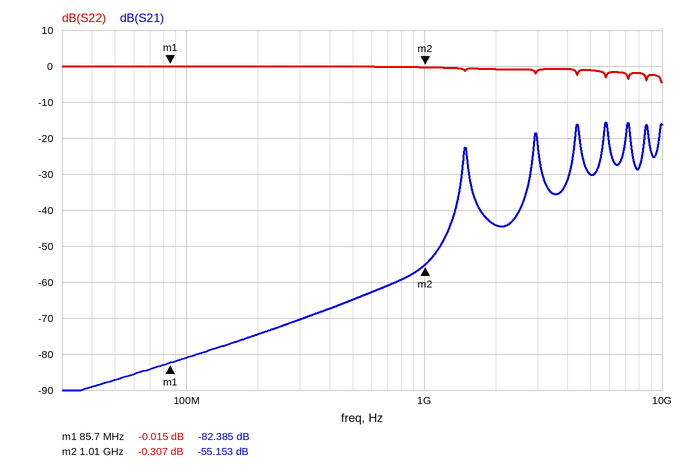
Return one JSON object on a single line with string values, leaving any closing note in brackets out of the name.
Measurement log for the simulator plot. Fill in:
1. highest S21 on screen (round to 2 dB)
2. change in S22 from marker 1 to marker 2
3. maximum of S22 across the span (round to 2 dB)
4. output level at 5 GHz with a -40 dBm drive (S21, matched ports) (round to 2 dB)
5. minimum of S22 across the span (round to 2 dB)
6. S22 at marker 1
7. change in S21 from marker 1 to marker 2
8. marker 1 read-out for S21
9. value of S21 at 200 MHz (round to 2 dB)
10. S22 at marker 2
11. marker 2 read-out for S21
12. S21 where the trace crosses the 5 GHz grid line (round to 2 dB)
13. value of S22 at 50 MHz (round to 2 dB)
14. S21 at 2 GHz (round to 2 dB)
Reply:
{"highest S21 on screen": "-16 dB", "change in S22 from marker 1 to marker 2": "-0.292 dB", "maximum of S22 across the span": "0 dB", "output level at 5 GHz with a -40 dBm drive (S21, matched ports)": "-70 dBm", "minimum of S22 across the span": "-4 dB", "S22 at marker 1": "-0.015 dB", "change in S21 from marker 1 to marker 2": "27.232 dB", "marker 1 read-out for S21": "-82.385 dB", "value of S21 at 200 MHz": "-74 dB", "S22 at marker 2": "-0.307 dB", "marker 2 read-out for S21": "-55.153 dB", "S21 where the trace crosses the 5 GHz grid line": "-30 dB", "value of S22 at 50 MHz": "0 dB", "S21 at 2 GHz": "-44 dB"}
